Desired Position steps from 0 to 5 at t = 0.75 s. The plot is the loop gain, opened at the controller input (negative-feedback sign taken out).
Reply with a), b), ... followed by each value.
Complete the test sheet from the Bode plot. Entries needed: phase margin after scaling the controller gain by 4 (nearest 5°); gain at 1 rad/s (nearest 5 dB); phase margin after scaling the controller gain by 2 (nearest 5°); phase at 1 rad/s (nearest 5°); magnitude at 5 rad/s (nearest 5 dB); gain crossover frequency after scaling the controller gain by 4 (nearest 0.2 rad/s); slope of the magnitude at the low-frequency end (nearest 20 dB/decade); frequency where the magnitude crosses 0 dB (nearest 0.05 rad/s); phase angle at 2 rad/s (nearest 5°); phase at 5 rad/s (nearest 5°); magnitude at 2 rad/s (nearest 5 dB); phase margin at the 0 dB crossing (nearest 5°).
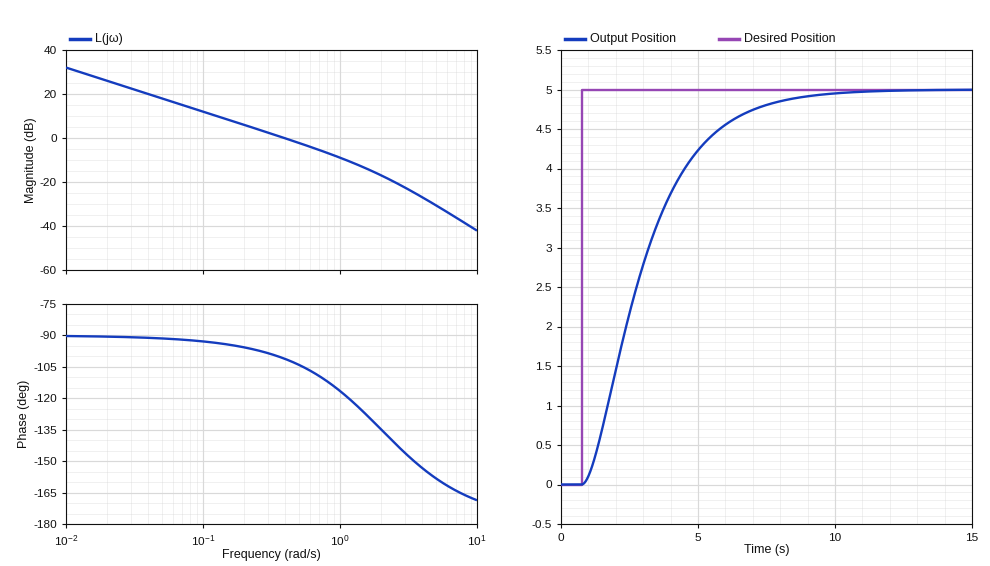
a) 55°
b) -10 dB
c) 70°
d) -115°
e) -30 dB
f) 1.4 rad/s
g) -20 dB/decade
h) 0.40 rad/s
i) -135°
j) -160°
k) -15 dB
l) 80°
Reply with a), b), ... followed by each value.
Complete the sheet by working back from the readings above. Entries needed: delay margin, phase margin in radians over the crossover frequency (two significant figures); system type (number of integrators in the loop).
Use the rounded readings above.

a) 3.5 s
b) 1
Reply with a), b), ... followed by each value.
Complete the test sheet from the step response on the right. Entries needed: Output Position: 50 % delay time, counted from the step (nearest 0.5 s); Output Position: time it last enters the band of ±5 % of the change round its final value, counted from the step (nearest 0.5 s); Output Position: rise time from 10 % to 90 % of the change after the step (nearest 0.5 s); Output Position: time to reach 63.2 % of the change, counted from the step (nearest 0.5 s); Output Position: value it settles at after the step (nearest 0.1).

a) 2.0 s
b) 6.5 s
c) 4.5 s
d) 2.5 s
e) 5.0
